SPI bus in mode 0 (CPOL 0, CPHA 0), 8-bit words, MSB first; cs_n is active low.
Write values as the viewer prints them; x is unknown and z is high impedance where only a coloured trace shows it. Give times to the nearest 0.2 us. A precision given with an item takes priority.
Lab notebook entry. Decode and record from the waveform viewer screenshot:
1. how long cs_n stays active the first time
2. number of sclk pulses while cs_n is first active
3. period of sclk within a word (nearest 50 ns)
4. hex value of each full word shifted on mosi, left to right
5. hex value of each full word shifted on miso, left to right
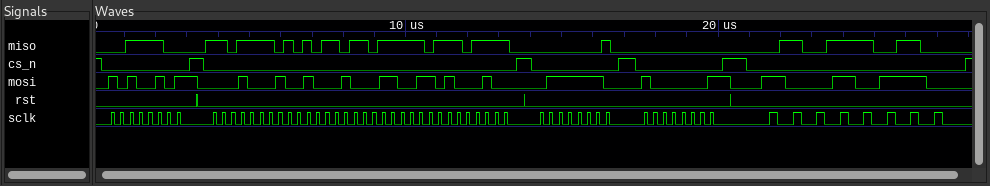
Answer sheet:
2.8 us
8
300 ns
A5, 11, 22, 33, 44, 7E, 81, 96
3C, DE, AD, BE, EF, 01, 00, 5A
